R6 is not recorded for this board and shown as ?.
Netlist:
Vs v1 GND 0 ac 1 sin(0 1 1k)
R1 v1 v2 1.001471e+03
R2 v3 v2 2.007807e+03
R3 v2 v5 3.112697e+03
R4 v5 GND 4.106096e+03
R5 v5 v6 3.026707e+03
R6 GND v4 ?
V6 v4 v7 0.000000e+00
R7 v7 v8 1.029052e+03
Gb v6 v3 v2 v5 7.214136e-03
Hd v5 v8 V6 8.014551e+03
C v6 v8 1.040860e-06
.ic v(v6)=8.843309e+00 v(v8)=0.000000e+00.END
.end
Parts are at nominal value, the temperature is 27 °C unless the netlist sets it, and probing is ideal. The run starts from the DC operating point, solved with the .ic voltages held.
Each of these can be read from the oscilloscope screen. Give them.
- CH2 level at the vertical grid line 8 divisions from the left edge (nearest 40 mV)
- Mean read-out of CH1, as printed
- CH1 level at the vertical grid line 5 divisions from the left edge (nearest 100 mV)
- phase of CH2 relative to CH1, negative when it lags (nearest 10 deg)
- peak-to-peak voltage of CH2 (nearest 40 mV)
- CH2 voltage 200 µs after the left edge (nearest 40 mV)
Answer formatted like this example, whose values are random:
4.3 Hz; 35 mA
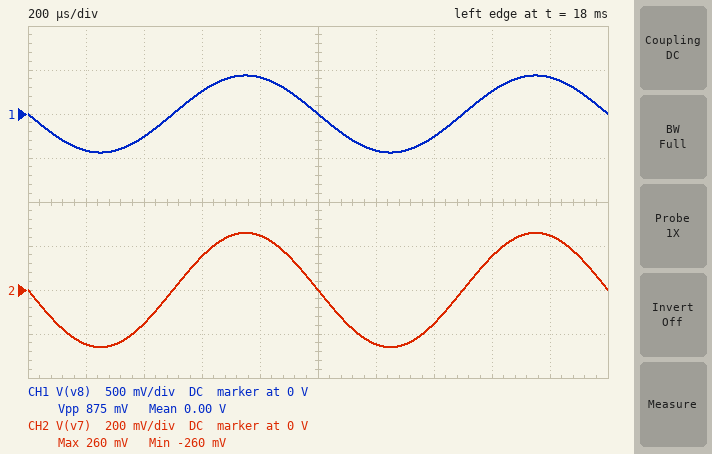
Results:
160 mV; 0.00 V; 0 V; 0 deg; 520 mV; -240 mV
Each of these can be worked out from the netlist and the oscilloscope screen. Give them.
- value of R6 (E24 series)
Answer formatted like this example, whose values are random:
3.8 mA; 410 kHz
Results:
1.5 kΩ
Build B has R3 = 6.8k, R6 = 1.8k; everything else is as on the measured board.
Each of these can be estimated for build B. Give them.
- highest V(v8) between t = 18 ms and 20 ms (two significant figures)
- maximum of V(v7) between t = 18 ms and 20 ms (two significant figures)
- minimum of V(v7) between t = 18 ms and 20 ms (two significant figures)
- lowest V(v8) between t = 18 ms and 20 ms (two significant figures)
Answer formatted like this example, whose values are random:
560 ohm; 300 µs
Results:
520 mV; 330 mV; -330 mV; -520 mV
